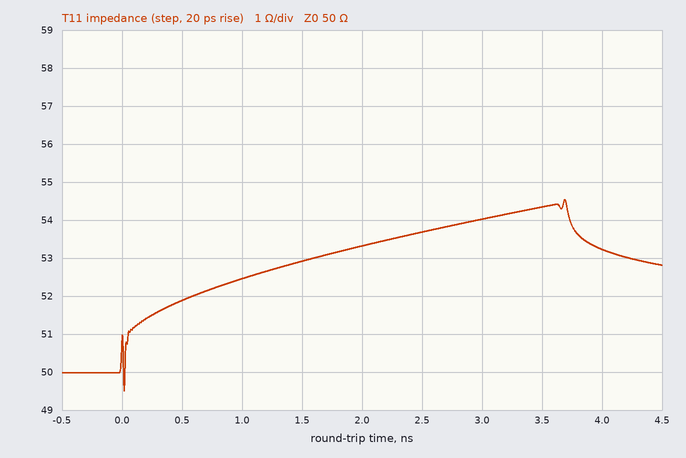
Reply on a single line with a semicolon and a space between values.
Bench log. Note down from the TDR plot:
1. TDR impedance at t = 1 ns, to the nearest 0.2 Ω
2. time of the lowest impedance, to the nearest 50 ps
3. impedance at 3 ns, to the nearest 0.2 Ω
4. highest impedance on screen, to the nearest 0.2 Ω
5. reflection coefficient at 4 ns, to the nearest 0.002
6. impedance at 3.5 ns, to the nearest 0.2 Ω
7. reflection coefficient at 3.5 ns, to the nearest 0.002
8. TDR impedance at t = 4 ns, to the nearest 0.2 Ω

52.4 Ω; 0 ps; 54.0 Ω; 54.6 Ω; +0.032; 54.4 Ω; +0.042; 53.2 Ω
